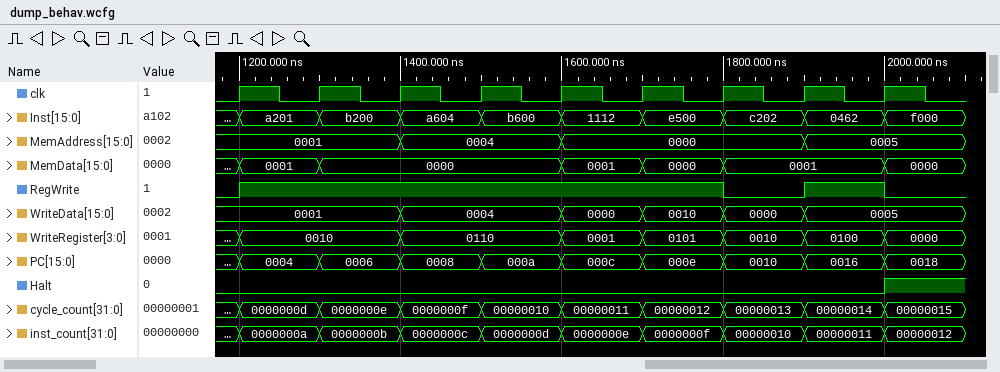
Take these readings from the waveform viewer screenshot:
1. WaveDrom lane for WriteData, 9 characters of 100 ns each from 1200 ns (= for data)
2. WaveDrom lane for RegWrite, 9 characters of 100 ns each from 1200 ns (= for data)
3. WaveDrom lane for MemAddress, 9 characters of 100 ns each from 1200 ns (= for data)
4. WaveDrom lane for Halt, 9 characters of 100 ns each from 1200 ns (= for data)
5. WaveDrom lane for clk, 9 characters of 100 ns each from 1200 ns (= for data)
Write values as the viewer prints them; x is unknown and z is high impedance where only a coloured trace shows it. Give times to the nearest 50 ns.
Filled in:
{name: 'WriteData', wave: '=.=.====.', data: '0001 0004 0000 0010 0000 0005'}
{name: 'RegWrite', wave: '1.....010'}
{name: 'MemAddress', wave: '=.=.=..=.', data: '0001 0004 0000 0005'}
{name: 'Halt', wave: '0.......1'}
{name: 'clk', wave: 'p........'}
